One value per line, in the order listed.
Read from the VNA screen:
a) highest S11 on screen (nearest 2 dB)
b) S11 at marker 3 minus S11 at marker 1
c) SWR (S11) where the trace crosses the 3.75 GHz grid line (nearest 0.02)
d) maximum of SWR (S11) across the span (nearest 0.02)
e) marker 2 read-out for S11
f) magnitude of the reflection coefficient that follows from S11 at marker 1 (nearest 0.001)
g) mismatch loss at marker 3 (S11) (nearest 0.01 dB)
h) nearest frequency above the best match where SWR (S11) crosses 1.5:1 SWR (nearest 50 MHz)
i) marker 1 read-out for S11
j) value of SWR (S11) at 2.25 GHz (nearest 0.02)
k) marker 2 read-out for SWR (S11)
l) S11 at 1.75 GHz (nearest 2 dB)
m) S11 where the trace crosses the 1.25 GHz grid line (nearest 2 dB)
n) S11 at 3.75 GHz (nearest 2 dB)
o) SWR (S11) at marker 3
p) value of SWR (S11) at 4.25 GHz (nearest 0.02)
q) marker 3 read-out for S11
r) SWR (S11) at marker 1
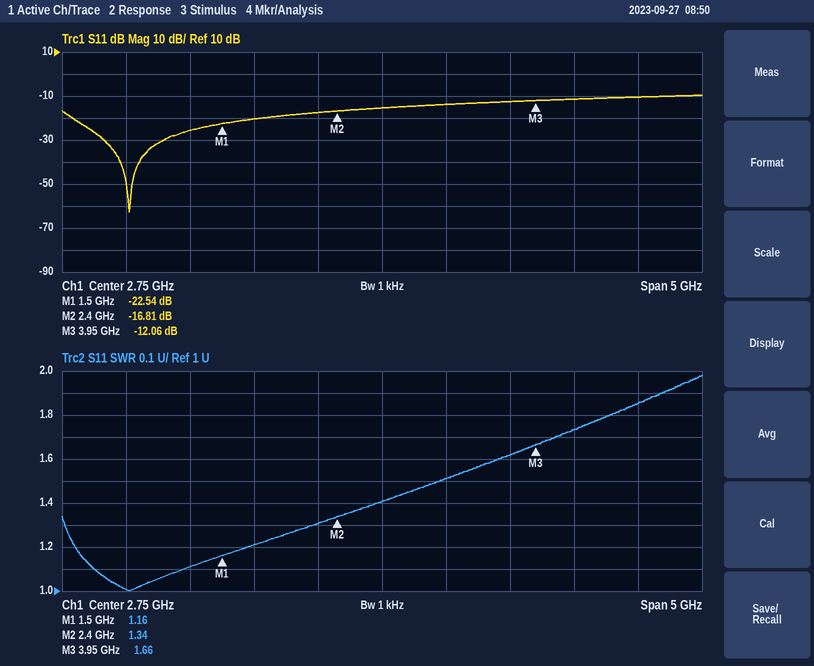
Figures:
-10 dB
10.48 dB
1.62
1.98
-16.81 dB
0.075
0.28 dB
3.20 GHz
-22.54 dB
1.30
1.34
-20 dB
-26 dB
-12 dB
1.66
1.74
-12.06 dB
1.16
